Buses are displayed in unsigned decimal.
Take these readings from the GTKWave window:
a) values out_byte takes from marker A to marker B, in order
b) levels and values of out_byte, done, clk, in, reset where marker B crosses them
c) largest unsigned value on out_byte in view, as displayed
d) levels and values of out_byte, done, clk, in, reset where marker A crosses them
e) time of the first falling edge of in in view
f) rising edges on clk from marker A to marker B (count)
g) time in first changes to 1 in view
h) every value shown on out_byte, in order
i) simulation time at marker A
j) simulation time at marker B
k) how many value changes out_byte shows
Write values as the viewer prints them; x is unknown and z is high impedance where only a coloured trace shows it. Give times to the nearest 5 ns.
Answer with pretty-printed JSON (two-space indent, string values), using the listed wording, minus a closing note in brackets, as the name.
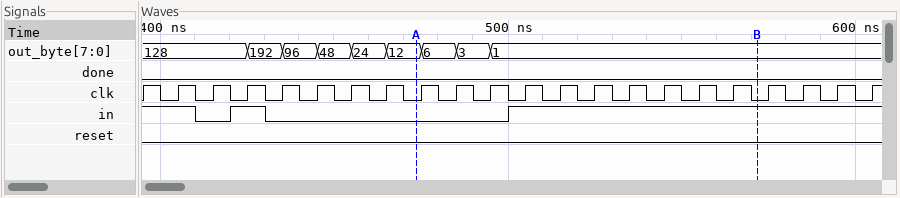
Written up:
{
  "values out_byte takes from marker A to marker B, in order": "12, 6, 3, 1",
  "levels and values of out_byte, done, clk, in, reset where marker B crosses them": "out_byte=1, done=0, clk=0, in=1, reset=0",
  "largest unsigned value on out_byte in view, as displayed": "192",
  "levels and values of out_byte, done, clk, in, reset where marker A crosses them": "out_byte=12, done=0, clk=0, in=0, reset=0",
  "time of the first falling edge of in in view": "410 ns",
  "rising edges on clk from marker A to marker B": "10",
  "time in first changes to 1 in view": "420 ns",
  "every value shown on out_byte, in order": "128, 192, 96, 48, 24, 12, 6, 3, 1",
  "simulation time at marker A": "475 ns",
  "simulation time at marker B": "570 ns",
  "how many value changes out_byte shows": "8"
}
